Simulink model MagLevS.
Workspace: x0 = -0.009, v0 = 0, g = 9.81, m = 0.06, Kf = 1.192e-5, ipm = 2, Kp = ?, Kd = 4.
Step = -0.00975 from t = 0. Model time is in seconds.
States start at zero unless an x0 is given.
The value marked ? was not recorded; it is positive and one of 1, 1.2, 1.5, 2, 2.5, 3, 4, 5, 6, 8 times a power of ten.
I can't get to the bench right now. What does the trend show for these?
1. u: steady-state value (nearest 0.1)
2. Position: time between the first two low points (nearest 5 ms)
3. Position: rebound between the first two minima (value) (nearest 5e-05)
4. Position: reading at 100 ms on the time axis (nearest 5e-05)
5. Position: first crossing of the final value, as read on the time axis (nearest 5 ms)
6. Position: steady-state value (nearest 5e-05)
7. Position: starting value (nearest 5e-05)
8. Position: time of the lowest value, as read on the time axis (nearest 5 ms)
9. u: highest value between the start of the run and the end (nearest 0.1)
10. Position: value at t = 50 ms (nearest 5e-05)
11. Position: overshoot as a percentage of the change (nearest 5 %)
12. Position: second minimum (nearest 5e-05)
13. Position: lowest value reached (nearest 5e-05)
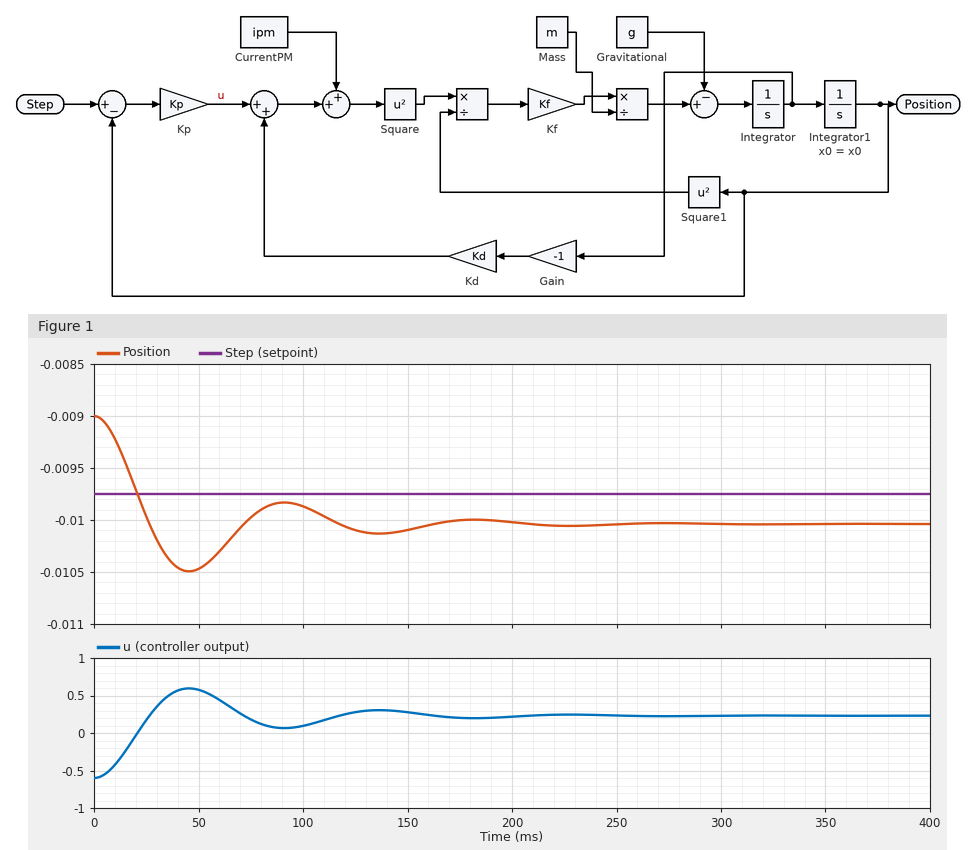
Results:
0.2
90 ms
-0.00985
-0.00985
25 ms
-0.01005
-0.00900
45 ms
0.6
-0.01045
45 %
-0.01015
-0.01050
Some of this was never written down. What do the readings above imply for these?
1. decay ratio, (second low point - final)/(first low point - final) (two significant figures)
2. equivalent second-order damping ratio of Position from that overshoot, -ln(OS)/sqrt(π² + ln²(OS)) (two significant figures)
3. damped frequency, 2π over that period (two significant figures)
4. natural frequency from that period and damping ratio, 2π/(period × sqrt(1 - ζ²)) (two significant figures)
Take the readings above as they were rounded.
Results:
0.22
0.25
0.070 rad/ms
0.072 rad/ms
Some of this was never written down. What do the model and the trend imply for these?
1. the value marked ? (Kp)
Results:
800
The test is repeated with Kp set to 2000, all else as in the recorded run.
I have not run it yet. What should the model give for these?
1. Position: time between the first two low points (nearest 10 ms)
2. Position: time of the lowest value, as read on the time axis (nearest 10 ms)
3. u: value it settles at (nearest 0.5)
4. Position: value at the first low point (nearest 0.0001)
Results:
50 ms
30 ms
0.0
-0.0103
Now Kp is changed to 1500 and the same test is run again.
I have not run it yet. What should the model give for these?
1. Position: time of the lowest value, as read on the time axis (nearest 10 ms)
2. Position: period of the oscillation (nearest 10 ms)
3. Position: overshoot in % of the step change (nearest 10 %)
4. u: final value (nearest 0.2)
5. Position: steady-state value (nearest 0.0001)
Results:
30 ms
60 ms
50 %
0.2
-0.0099
